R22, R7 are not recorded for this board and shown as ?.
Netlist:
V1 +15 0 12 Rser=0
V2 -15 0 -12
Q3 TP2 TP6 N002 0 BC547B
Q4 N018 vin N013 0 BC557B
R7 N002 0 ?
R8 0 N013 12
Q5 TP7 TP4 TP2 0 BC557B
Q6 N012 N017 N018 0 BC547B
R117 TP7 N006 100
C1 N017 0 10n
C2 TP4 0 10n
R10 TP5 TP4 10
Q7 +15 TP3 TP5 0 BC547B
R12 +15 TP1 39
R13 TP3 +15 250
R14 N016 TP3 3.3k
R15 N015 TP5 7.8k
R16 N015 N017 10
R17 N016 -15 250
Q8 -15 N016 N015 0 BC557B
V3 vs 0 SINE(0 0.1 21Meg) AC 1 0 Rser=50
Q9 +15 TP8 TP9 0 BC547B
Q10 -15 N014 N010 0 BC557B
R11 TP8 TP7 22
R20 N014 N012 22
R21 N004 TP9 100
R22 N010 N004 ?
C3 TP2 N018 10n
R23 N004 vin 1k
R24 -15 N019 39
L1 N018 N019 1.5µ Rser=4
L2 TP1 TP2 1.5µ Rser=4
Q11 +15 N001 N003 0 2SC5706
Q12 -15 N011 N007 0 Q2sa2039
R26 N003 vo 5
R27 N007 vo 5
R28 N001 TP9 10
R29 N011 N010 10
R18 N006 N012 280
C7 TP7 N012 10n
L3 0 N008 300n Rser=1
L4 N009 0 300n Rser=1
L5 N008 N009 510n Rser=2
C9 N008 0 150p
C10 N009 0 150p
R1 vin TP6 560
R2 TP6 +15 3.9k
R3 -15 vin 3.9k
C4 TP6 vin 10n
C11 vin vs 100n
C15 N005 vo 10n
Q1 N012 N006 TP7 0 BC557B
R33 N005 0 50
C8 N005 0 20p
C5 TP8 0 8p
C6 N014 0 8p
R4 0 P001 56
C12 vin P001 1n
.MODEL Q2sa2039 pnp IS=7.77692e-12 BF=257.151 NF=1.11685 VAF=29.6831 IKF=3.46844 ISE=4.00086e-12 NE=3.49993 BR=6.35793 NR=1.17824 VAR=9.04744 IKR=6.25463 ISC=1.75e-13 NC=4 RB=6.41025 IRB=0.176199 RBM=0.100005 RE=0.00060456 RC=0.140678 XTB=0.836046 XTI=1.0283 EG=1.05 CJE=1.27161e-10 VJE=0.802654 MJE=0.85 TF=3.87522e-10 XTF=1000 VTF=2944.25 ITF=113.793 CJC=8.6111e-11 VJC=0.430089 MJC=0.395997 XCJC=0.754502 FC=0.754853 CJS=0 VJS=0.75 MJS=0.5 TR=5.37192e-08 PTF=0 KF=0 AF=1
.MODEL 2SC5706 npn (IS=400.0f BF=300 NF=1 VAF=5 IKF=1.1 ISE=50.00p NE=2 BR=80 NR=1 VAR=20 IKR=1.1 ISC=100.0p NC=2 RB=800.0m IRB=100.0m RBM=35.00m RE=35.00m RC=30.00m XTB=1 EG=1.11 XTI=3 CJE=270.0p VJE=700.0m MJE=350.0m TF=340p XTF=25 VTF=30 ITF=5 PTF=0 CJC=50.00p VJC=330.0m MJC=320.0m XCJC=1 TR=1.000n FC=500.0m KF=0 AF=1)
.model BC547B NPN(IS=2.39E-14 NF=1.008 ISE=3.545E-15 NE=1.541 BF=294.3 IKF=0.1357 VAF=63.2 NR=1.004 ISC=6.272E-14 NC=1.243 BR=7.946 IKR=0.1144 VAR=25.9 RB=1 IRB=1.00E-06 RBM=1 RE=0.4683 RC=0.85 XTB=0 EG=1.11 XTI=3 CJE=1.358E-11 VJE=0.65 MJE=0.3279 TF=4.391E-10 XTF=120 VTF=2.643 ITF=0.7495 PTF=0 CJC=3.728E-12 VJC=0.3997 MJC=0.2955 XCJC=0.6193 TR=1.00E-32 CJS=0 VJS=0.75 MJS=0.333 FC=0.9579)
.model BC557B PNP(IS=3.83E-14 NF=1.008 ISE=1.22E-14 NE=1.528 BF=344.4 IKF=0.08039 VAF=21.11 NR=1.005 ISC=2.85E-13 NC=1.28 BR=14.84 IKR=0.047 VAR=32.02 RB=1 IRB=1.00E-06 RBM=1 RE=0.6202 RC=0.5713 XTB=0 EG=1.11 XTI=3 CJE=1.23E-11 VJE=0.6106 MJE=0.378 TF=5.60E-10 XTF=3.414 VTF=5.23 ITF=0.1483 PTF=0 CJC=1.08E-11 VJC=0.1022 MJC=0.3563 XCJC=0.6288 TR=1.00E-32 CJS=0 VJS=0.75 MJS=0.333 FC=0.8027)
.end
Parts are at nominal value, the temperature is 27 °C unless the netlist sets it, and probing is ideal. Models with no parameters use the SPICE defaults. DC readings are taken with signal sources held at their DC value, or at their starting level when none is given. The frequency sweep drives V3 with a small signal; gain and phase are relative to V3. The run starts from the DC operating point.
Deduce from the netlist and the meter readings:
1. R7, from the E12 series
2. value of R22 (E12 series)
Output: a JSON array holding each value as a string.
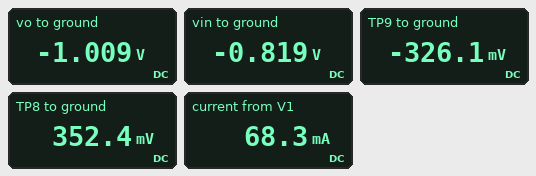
["5.6 Ω", "180 Ω"]
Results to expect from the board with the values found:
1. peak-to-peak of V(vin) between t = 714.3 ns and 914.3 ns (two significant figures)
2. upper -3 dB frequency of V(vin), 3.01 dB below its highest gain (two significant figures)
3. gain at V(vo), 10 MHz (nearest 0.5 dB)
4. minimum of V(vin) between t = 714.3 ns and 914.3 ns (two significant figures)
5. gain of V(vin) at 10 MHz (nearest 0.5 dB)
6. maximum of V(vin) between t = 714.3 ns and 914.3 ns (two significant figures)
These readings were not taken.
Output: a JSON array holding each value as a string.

["140 mV", "43 MHz", "27.0 dB", "-890 mV", "-14.0 dB", "-750 mV"]
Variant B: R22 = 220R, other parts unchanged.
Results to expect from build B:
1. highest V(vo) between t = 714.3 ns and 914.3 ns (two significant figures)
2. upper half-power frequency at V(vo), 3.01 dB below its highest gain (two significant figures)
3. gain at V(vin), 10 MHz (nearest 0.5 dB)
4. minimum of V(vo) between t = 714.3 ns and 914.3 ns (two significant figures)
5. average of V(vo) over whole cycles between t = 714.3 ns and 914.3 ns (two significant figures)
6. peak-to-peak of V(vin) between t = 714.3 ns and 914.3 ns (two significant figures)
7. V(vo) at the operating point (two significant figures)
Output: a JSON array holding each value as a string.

["1.6 V", "33 MHz", "-13.5 dB", "-4.1 V", "-1.2 V", "150 mV", "-1.1 V"]
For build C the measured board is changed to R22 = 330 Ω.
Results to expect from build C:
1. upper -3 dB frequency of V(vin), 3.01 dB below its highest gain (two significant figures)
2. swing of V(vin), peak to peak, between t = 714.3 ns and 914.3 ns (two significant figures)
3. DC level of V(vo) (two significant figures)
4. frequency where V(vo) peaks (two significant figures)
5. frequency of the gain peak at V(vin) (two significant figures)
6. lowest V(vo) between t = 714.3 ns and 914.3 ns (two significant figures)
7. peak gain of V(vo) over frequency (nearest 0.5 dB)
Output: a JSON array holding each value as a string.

["42 MHz", "160 mV", "-1.2 V", "23 MHz", "28 MHz", "-4.2 V", "29.5 dB"]
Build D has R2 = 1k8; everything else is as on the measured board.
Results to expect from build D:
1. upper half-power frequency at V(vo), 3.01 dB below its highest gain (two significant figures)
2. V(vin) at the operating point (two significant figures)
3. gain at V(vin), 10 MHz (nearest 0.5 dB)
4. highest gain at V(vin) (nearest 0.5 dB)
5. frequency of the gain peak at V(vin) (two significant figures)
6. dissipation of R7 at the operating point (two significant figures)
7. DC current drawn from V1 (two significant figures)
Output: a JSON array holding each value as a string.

["620 kHz", "-1.2 V", "-10.5 dB", "-1.5 dB", "590 kHz", "94 mW", "140 mA"]
